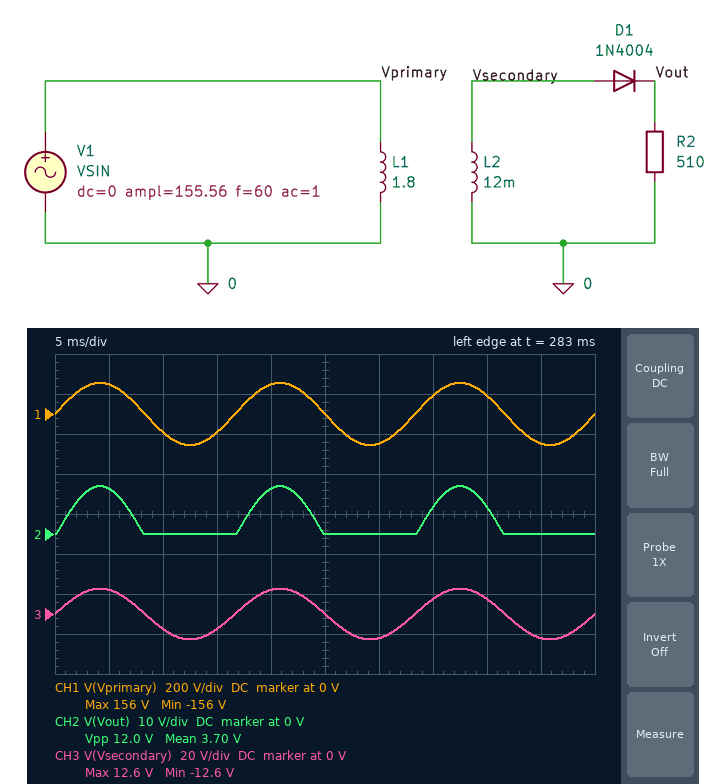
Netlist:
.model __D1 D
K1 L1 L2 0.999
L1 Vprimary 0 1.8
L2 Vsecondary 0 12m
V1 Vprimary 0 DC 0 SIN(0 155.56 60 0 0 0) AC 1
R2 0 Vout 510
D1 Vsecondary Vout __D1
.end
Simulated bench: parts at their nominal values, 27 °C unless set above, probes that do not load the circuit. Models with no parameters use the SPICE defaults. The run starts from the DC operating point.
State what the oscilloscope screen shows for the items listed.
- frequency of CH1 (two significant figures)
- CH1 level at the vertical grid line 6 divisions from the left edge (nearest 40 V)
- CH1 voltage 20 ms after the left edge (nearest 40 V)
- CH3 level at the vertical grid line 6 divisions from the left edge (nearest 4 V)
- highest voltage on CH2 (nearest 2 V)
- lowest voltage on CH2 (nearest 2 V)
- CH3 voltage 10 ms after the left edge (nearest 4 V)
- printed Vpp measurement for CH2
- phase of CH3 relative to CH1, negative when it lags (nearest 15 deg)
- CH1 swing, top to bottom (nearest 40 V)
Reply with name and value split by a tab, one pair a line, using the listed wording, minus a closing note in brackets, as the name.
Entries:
frequency of CH1	60 Hz
CH1 level at the vertical grid line 6 divisions from the left edge	-160 V
CH1 voltage 20 ms after the left edge	160 V
CH3 level at the vertical grid line 6 divisions from the left edge	-12 V
highest voltage on CH2	12 V
lowest voltage on CH2	0 V
CH3 voltage 10 ms after the left edge	-8 V
printed Vpp measurement for CH2	12.0 V
phase of CH3 relative to CH1, negative when it lags	0 deg
CH1 swing, top to bottom	320 V
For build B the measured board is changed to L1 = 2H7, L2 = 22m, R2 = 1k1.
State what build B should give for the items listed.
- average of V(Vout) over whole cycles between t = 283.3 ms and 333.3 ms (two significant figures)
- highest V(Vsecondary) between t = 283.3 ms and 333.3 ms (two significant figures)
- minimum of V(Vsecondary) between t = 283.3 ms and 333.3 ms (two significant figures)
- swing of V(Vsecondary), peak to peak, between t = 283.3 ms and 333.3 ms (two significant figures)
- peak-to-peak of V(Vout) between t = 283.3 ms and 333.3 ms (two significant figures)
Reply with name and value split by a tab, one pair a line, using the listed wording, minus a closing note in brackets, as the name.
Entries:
average of V(Vout) over whole cycles between t = 283.3 ms and 333.3 ms	4.1 V
highest V(Vsecondary) between t = 283.3 ms and 333.3 ms	14 V
minimum of V(Vsecondary) between t = 283.3 ms and 333.3 ms	-14 V
swing of V(Vsecondary), peak to peak, between t = 283.3 ms and 333.3 ms	28 V
peak-to-peak of V(Vout) between t = 283.3 ms and 333.3 ms	13 V
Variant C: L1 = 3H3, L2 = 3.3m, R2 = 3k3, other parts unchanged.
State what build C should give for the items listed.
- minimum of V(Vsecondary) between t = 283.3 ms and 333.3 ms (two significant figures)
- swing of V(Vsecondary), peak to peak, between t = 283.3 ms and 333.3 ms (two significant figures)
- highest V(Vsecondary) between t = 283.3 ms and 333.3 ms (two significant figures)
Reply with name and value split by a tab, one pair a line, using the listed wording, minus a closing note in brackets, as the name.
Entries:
minimum of V(Vsecondary) between t = 283.3 ms and 333.3 ms	-4.9 V
swing of V(Vsecondary), peak to peak, between t = 283.3 ms and 333.3 ms	9.8 V
highest V(Vsecondary) between t = 283.3 ms and 333.3 ms	4.9 V
